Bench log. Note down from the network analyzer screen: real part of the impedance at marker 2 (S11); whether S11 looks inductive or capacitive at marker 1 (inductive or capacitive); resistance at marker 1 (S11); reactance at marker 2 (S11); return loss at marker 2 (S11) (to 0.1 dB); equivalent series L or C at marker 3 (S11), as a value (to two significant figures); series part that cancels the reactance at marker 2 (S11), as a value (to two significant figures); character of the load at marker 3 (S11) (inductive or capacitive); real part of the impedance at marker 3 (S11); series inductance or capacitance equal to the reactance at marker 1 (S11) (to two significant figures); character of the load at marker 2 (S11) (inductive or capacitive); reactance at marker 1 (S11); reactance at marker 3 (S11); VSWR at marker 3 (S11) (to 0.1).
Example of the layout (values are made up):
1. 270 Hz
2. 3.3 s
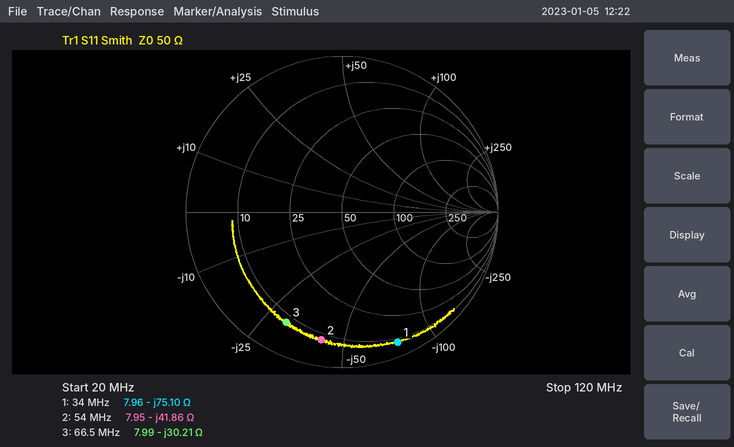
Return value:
1. 7.95 Ω
2. capacitive
3. 7.96 Ω
4. -41.86 Ω
5. 1.6 dB
6. 79 pF
7. 120 nH
8. capacitive
9. 7.99 Ω
10. 62 pF
11. capacitive
12. -75.10 Ω
13. -30.21 Ω
14. 8.6
